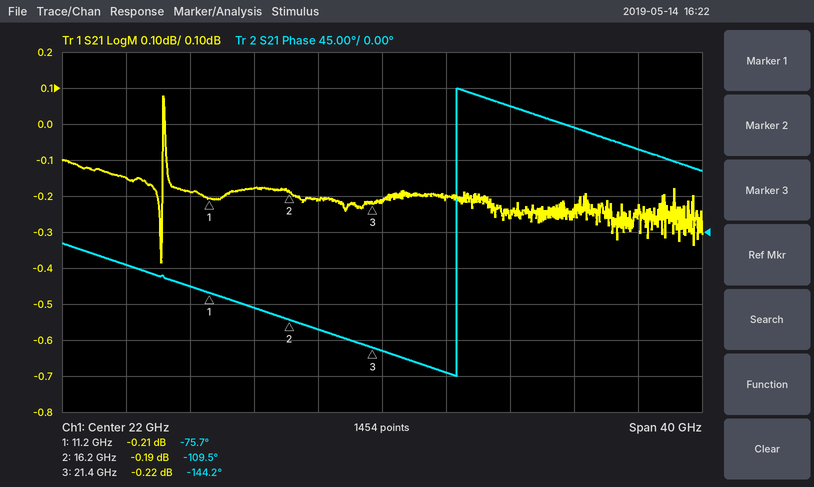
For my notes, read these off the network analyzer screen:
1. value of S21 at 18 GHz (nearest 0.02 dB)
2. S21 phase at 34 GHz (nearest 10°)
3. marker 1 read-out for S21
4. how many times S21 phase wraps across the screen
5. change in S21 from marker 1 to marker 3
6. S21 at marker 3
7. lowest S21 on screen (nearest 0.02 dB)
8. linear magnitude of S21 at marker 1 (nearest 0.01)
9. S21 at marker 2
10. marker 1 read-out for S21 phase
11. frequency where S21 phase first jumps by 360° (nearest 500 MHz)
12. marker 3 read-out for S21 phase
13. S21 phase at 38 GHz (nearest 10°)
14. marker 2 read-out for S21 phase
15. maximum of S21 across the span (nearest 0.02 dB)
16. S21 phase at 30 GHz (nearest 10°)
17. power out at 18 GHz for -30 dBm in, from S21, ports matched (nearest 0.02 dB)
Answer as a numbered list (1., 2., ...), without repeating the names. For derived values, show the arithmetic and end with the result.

1. -0.20 dB
2. 130°
3. -0.21 dB
4. 1
5. -0.22 − (-0.21) = -0.01 dB
6. -0.22 dB
7. -0.38 dB
8. 10^(-0.21/20) ≈ 0.98
9. -0.19 dB
10. -75.7°
11. 26.5 GHz
12. -144.2°
13. 100°
14. -109.5°
15. 0.08 dB
16. 160°
17. -30 dBm + (-0.20 dB) = -30.20 dBm
